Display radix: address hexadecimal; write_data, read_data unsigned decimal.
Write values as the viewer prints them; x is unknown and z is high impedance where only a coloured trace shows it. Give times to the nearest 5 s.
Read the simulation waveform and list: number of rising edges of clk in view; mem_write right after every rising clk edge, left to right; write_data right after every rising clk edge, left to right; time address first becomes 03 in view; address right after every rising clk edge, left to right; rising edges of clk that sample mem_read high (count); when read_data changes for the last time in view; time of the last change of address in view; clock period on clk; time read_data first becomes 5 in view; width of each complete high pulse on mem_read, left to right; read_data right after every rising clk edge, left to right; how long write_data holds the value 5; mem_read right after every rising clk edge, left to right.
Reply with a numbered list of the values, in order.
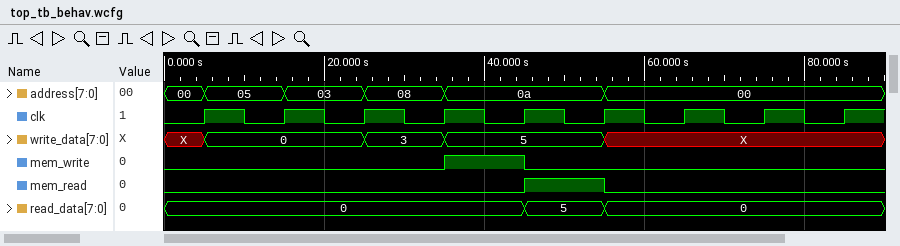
1. 9
2. 0 0 0 1 0 0 0 0 0
3. 0, 0, 3, 5, 5, X, X, X, X
4. 15 s
5. 05, 03, 08, 0a, 0a, 00, 00, 00, 00
6. 1
7. 55 s
8. 55 s
9. 10 s
10. 45 s
11. 10 s
12. 0, 0, 0, 0, 5, 0, 0, 0, 0
13. 20 s
14. 0 0 0 0 1 0 0 0 0
